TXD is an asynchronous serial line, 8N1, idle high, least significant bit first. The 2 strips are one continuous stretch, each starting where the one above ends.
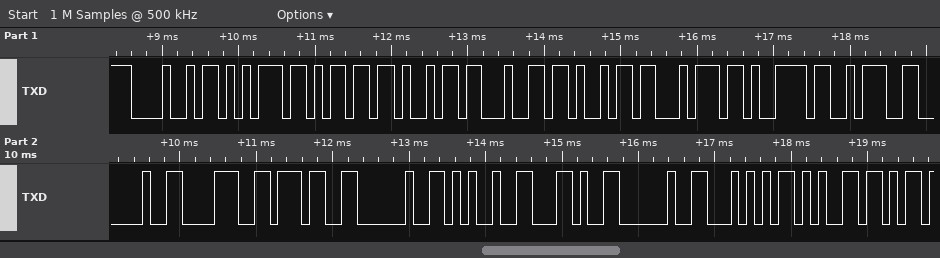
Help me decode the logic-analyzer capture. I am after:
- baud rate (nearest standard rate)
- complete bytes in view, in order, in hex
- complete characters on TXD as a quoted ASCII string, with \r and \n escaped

9600 baud
48 75 6D 69 64 69 74 79 3A 20 38 37 20 25 2C 20 54 65
"Humidity: 87 %, Te"
